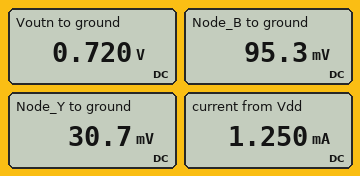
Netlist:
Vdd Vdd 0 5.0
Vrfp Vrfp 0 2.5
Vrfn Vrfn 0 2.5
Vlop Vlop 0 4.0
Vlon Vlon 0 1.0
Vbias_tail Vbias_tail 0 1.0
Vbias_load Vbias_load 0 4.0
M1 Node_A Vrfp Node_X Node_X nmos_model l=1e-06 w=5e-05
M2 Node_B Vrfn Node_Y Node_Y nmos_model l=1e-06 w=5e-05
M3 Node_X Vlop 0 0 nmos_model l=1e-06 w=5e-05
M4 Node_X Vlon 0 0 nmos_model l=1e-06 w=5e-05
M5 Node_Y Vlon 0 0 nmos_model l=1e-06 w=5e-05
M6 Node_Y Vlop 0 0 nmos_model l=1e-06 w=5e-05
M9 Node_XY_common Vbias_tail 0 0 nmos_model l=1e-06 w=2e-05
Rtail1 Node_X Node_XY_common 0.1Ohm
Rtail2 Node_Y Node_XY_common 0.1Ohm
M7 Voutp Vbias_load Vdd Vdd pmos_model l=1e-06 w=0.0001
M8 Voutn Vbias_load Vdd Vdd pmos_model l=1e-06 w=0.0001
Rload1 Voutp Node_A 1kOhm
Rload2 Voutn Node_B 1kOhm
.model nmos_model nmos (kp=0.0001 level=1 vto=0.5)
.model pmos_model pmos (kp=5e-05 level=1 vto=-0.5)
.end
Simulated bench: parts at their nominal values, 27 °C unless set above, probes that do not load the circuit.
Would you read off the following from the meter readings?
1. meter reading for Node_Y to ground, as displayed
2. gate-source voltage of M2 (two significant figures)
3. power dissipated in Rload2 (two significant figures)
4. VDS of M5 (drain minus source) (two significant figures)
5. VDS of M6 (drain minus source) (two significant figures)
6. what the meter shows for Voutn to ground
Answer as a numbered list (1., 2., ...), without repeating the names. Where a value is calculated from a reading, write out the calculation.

1. 30.7 mV
2. 2.5 V - 30.7 mV = 2.5 V
3. (720 mV - 95.3 mV)^2 / 1 kΩ = 390 µW
4. 30.7 mV = 31 mV
5. 30.7 mV = 31 mV
6. 0.720 V
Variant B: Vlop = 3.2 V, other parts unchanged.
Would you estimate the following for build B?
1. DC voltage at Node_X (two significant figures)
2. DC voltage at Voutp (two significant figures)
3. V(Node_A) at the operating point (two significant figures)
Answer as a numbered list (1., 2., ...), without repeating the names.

1. 38 mV
2. 730 mV
3. 100 mV
